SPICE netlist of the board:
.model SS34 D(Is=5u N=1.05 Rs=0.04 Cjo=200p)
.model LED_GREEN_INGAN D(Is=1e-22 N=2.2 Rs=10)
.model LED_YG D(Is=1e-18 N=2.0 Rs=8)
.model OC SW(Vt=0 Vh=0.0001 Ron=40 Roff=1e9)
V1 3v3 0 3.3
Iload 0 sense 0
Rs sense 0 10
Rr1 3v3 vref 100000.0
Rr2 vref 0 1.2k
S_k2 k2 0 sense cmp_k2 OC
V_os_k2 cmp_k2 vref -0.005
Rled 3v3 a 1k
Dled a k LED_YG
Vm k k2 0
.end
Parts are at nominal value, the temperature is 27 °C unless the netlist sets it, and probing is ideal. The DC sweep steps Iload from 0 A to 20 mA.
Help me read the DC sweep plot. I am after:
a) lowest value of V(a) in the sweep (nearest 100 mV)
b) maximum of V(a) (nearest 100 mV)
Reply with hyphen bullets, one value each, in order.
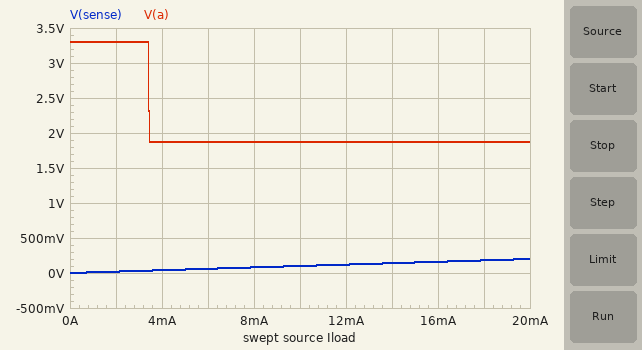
- 1.9 V
- 3.3 V
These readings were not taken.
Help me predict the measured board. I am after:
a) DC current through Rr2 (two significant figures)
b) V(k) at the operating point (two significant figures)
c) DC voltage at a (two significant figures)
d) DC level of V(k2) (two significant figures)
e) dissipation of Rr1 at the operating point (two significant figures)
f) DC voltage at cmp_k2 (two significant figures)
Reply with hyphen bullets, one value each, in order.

- 33 µA
- 2.2 V
- 3.3 V
- 2.2 V
- 110 µW
- 34 mV
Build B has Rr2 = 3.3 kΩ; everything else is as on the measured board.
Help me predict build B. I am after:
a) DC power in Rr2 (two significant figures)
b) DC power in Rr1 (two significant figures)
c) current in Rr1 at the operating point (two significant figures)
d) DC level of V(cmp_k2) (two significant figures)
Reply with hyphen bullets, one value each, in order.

- 3.4 µW
- 100 µW
- 32 µA
- 100 mV
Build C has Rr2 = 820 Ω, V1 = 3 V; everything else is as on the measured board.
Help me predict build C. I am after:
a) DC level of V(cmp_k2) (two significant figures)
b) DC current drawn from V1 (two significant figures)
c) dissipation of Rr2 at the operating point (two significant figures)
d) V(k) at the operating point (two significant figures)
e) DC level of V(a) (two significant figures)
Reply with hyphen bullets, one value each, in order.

- 19 mV
- 30 µA
- 730 nW
- 1.9 V
- 3.0 V
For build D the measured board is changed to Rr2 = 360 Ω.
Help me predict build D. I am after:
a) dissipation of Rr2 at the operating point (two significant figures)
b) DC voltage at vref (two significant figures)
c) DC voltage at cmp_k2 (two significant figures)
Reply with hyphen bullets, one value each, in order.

- 390 nW
- 12 mV
- 6.8 mV
